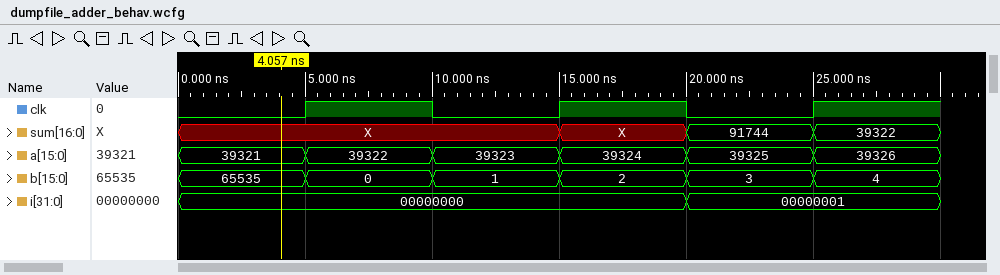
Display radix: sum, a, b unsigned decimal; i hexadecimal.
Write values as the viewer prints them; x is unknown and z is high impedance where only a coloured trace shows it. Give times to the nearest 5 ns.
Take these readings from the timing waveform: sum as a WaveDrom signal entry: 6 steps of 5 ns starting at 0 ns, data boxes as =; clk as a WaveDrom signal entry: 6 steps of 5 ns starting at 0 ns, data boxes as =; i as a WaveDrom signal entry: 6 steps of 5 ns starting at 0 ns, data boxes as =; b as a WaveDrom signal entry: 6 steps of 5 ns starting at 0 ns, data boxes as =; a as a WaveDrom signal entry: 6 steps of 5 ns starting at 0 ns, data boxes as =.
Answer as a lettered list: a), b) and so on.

a) {name: 'sum', wave: 'x..===', data: 'X 91744 39322'}
b) {name: 'clk', wave: '010101'}
c) {name: 'i', wave: '=...=.', data: '00000000 00000001'}
d) {name: 'b', wave: '======', data: '65535 0 1 2 3 4'}
e) {name: 'a', wave: '======', data: '39321 39322 39323 39324 39325 39326'}
